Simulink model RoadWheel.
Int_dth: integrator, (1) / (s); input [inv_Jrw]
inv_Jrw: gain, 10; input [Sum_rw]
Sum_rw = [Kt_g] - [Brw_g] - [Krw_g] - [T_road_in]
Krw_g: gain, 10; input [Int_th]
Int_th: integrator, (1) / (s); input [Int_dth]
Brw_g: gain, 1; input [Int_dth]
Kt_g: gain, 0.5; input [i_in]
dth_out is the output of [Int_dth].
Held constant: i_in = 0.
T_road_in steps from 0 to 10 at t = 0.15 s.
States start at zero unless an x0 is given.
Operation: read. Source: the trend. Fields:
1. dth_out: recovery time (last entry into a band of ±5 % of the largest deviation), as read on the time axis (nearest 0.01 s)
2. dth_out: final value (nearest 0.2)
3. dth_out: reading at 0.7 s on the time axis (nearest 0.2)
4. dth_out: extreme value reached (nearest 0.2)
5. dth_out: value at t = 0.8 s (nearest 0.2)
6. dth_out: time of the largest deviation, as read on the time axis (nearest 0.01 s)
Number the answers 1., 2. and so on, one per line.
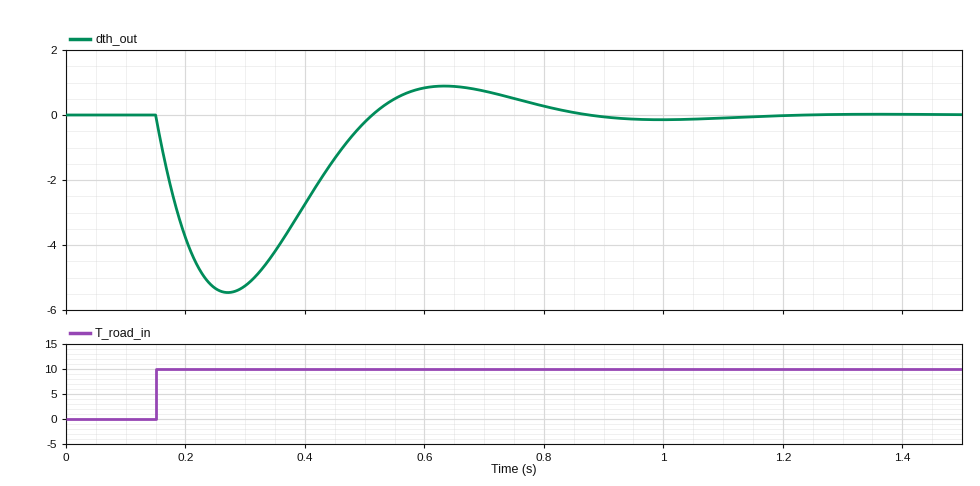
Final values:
1. 0.80 s
2. 0.0
3. 0.8
4. -5.4
5. 0.2
6. 0.27 s
